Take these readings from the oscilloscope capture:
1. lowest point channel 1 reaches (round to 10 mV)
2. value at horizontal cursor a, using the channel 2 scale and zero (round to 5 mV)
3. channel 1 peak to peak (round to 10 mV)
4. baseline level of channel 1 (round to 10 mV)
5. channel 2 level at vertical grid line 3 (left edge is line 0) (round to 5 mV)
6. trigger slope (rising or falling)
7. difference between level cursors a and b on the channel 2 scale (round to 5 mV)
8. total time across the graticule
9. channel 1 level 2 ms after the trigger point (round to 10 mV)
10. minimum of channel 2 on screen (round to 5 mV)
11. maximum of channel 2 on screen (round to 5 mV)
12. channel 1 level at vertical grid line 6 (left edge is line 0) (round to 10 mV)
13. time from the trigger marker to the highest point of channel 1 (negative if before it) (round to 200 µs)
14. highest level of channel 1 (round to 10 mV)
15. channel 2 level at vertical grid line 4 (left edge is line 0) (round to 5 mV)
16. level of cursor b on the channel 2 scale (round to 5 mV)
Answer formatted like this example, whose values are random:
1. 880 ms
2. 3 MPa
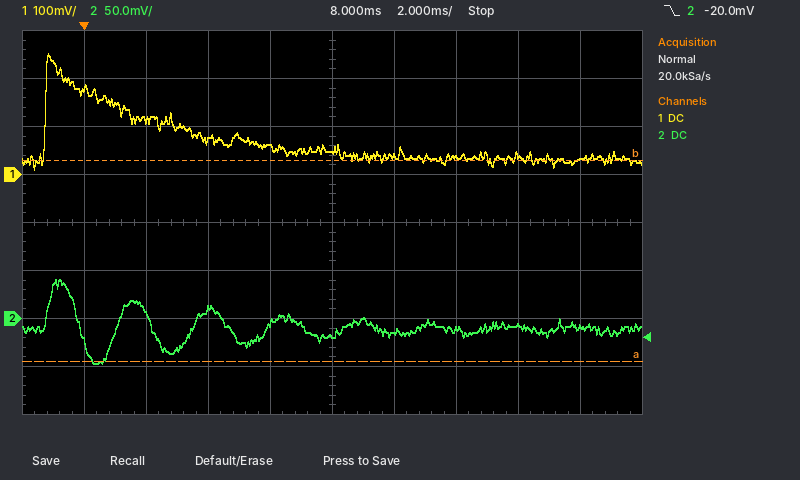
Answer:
1. 10 mV
2. -45 mV
3. 240 mV
4. 40 mV
5. 10 mV
6. falling
7. 210 mV
8. 20 ms
9. 110 mV
10. -45 mV
11. 40 mV
12. 40 mV
13. -1.2 ms
14. 250 mV
15. -5 mV
16. 165 mV
